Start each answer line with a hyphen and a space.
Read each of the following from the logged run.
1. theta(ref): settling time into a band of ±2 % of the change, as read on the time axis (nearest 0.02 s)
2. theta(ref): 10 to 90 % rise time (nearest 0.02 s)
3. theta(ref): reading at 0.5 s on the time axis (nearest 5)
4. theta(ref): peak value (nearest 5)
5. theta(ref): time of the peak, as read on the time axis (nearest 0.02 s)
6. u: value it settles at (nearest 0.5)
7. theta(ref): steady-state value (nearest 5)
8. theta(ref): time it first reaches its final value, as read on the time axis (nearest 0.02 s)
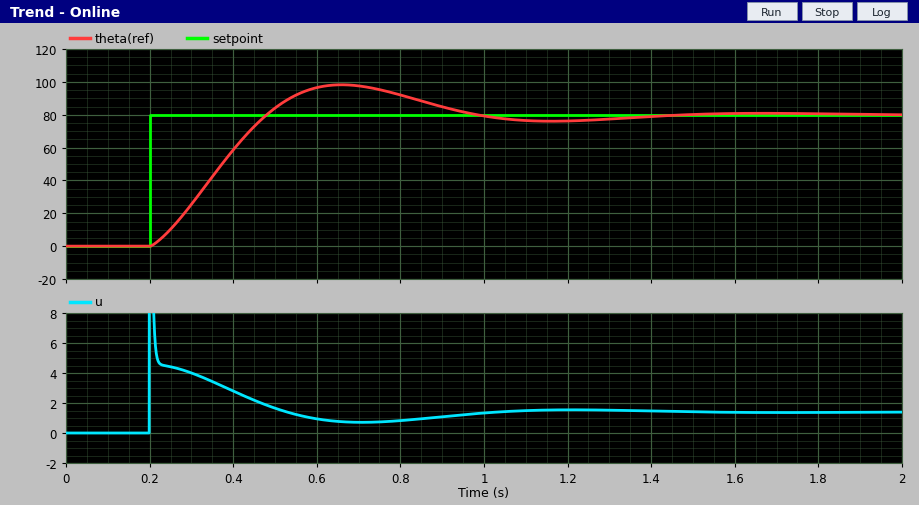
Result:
- 1.36 s
- 0.20 s
- 85
- 100
- 0.66 s
- 1.5
- 80
- 0.48 s
